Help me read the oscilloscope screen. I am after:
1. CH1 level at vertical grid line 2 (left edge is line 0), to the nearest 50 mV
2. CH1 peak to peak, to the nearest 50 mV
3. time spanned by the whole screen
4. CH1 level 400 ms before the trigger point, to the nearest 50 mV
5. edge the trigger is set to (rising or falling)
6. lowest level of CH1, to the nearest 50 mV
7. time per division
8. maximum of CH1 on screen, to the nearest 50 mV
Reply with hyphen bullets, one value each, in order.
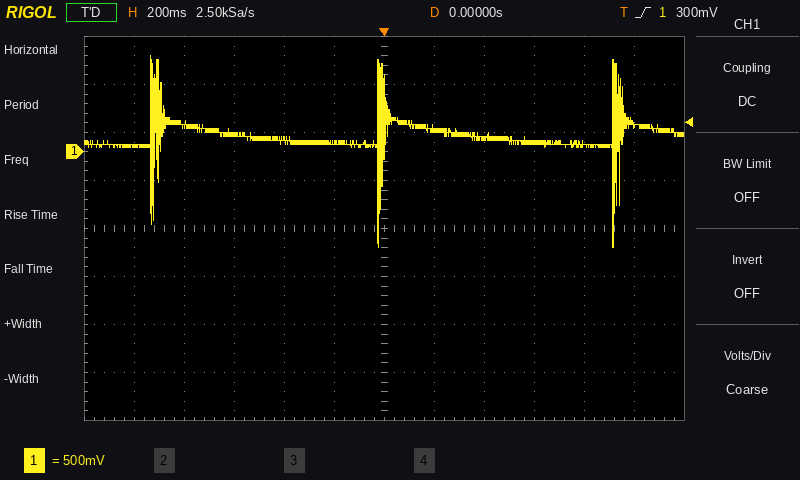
- 300 mV
- 2.00 V
- 2.4 s
- 100 mV
- rising
- -1.00 V
- 200 ms
- 1.00 V
